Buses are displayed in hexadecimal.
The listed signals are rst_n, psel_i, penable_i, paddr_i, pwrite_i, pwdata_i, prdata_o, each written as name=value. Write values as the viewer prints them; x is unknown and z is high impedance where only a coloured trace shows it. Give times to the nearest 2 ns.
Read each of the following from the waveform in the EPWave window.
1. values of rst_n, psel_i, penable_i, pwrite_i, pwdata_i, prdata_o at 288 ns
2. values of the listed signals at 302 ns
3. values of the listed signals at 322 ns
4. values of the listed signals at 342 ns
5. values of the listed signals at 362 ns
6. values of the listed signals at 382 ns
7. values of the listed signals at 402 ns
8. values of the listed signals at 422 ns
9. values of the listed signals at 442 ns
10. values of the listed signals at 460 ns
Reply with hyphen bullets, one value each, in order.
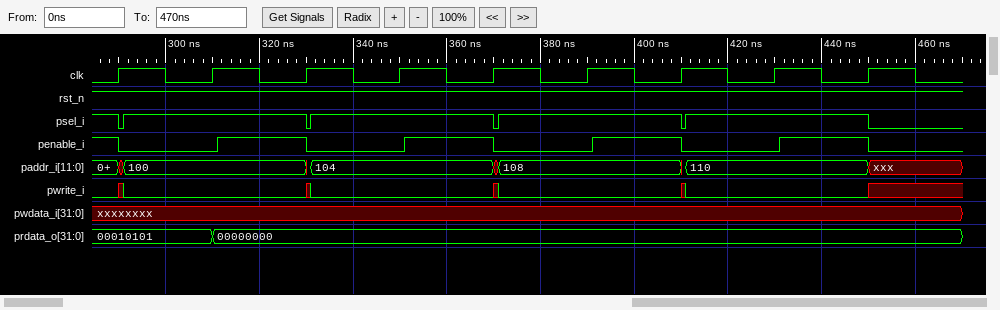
- rst_n=1, psel_i=1, penable_i=1, pwrite_i=0, pwdata_i=xxxxxxxx, prdata_o=00010101
- rst_n=1, psel_i=1, penable_i=0, paddr_i=100, pwrite_i=0, pwdata_i=xxxxxxxx, prdata_o=00010101
- rst_n=1, psel_i=1, penable_i=1, paddr_i=100, pwrite_i=0, pwdata_i=xxxxxxxx, prdata_o=00000000
- rst_n=1, psel_i=1, penable_i=0, paddr_i=104, pwrite_i=0, pwdata_i=xxxxxxxx, prdata_o=00000000
- rst_n=1, psel_i=1, penable_i=1, paddr_i=104, pwrite_i=0, pwdata_i=xxxxxxxx, prdata_o=00000000
- rst_n=1, psel_i=1, penable_i=0, paddr_i=108, pwrite_i=0, pwdata_i=xxxxxxxx, prdata_o=00000000
- rst_n=1, psel_i=1, penable_i=1, paddr_i=108, pwrite_i=0, pwdata_i=xxxxxxxx, prdata_o=00000000
- rst_n=1, psel_i=1, penable_i=0, paddr_i=110, pwrite_i=0, pwdata_i=xxxxxxxx, prdata_o=00000000
- rst_n=1, psel_i=1, penable_i=1, paddr_i=110, pwrite_i=0, pwdata_i=xxxxxxxx, prdata_o=00000000
- rst_n=1, psel_i=0, penable_i=0, paddr_i=xxx, pwrite_i=x, pwdata_i=xxxxxxxx, prdata_o=00000000
